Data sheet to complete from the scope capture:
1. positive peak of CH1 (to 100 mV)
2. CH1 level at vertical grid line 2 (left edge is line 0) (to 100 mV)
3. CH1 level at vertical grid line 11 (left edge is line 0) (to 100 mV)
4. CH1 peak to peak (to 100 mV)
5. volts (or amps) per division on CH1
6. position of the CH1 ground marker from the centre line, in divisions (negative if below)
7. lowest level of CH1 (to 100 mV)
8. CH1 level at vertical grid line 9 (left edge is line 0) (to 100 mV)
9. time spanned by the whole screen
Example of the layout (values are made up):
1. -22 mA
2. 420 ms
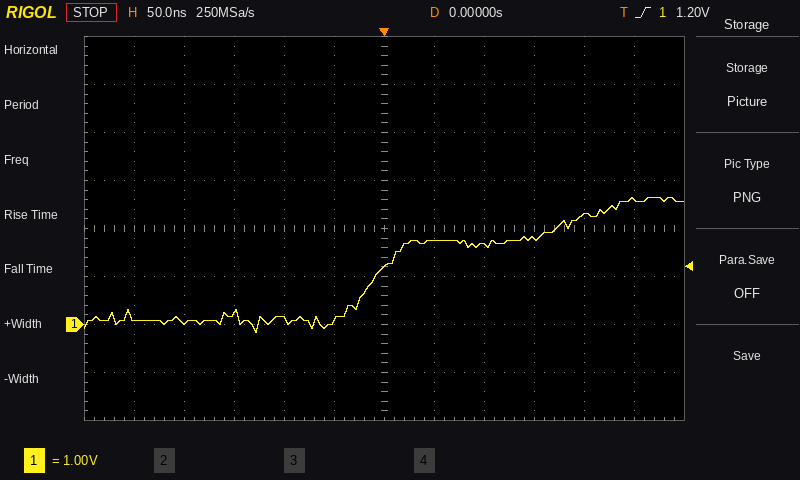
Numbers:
1. 2.6 V
2. 0.0 V
3. 2.6 V
4. 2.8 V
5. 1 V
6. -2.0 div
7. -200 mV
8. 1.8 V
9. 600 ns
